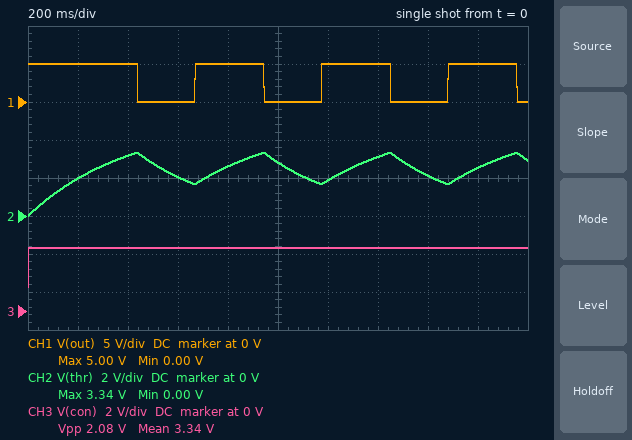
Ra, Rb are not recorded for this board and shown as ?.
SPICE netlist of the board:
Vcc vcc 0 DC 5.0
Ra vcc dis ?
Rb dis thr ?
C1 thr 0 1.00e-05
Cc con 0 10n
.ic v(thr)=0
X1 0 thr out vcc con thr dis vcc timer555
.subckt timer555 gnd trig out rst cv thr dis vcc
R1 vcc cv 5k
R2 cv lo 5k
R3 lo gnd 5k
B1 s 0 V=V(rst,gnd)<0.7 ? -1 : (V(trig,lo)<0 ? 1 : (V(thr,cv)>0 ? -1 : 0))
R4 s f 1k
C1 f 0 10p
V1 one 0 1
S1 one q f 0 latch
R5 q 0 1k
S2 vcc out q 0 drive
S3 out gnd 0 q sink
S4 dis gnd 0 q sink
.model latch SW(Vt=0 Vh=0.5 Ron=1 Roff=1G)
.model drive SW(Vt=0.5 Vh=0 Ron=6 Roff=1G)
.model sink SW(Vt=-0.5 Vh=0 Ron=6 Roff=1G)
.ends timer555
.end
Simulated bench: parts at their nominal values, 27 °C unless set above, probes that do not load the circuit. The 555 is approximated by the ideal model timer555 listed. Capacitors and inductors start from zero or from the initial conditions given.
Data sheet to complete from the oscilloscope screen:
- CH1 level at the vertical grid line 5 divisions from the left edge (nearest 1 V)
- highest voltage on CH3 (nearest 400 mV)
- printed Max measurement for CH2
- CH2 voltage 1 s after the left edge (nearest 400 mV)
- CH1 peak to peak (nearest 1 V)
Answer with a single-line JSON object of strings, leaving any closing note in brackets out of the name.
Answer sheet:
{"CH1 level at the vertical grid line 5 divisions from the left edge": "0 V", "highest voltage on CH3": "3.2 V", "printed Max measurement for CH2": "3.34 V", "CH2 voltage 1 s after the left edge": "2.8 V", "CH1 peak to peak": "5 V"}
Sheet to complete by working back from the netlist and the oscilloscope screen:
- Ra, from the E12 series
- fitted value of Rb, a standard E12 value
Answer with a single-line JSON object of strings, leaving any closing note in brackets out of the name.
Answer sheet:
{"Ra, from the E12 series": "6.8 kΩ", "fitted value of Rb, a standard E12 value": "33 kΩ"}
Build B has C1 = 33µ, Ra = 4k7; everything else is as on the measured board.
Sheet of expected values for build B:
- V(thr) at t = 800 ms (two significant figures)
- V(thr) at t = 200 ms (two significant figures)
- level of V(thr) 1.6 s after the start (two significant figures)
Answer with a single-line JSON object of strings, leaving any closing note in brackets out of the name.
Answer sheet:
{"V(thr) at t = 800 ms": "2.4 V", "V(thr) at t = 200 ms": "740 mV", "level of V(thr) 1.6 s after the start": "2.7 V"}
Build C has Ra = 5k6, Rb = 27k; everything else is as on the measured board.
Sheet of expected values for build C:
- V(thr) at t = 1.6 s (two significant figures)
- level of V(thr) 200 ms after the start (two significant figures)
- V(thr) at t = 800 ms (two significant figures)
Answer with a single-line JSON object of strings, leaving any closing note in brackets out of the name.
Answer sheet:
{"V(thr) at t = 1.6 s": "3.3 V", "level of V(thr) 200 ms after the start": "2.3 V", "V(thr) at t = 800 ms": "3.0 V"}
